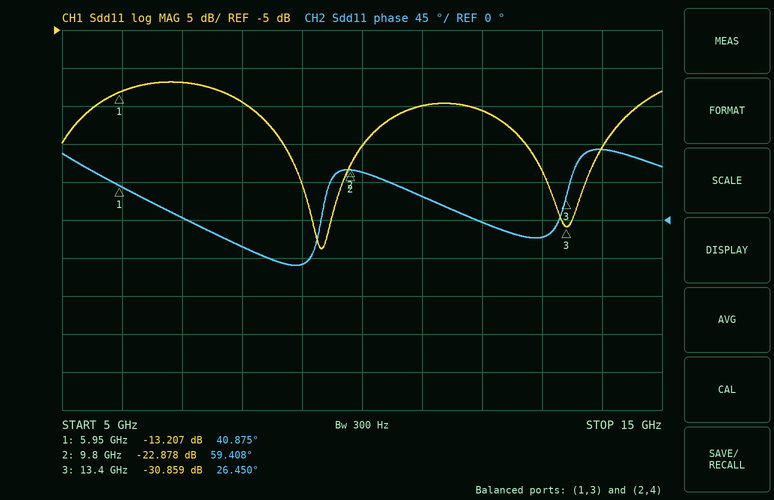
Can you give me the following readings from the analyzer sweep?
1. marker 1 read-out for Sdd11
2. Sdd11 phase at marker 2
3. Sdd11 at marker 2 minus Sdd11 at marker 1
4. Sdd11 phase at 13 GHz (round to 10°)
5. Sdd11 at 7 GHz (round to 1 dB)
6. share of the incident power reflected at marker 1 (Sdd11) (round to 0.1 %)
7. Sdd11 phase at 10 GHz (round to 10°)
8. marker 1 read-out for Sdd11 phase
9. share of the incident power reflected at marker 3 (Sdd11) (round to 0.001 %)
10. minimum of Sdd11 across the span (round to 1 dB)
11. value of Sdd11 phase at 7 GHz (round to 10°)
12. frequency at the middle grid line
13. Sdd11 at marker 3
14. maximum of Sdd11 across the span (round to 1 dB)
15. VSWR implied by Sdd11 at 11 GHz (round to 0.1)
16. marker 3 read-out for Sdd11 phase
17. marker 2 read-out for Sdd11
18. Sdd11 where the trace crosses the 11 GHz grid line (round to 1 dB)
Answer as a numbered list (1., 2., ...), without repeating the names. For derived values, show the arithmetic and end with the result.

1. -13.207 dB
2. 59.408°
3. -22.878 − (-13.207) = -9.671 dB
4. -20°
5. -12 dB
6. 10^(-13.207/10) ≈ 4.8 %
7. 60°
8. 40.875°
9. 10^(-30.859/10) ≈ 0.082 %
10. -34 dB
11. 0°
12. 10 GHz
13. -30.859 dB
14. -12 dB
15. |Γ| = 10^(-15/20) = 0.1778; VSWR = (1 + 0.1778)/(1 − 0.1778) ≈ 1.4
16. 26.450°
17. -22.878 dB
18. -15 dB
